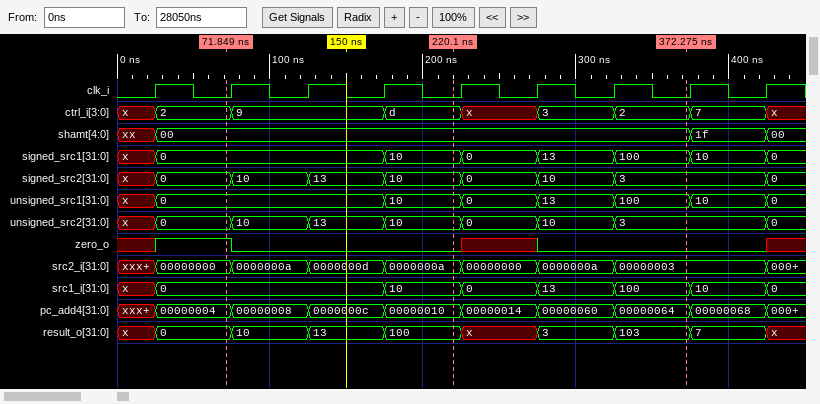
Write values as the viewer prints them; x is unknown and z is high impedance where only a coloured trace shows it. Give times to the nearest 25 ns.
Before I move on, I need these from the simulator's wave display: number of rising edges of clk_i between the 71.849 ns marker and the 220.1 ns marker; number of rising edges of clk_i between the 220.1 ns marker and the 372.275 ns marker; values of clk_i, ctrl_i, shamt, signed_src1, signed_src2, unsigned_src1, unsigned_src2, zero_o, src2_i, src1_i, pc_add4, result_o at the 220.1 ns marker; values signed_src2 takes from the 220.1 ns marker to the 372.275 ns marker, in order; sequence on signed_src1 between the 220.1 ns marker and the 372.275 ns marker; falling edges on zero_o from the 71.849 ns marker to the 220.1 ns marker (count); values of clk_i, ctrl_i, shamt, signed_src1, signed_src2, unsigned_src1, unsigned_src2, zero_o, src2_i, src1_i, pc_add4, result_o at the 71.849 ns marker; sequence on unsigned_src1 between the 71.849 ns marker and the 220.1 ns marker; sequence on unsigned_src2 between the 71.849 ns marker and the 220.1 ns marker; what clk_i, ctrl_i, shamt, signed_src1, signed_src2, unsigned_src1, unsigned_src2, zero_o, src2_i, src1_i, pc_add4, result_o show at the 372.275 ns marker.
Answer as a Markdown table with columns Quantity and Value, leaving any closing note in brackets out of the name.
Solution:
| Quantity | Value |
|---|---|
| number of rising edges of clk_i between the 71.849 ns marker and the 220.1 ns marker | 3 |
| number of rising edges of clk_i between the 220.1 ns marker and the 372.275 ns marker | 3 |
| values of clk_i, ctrl_i, shamt, signed_src1, signed_src2, unsigned_src1, unsigned_src2, zero_o, src2_i, src1_i, pc_add4, result_o at the 220.1 ns marker | clk_i=0, ctrl_i=d, shamt=00, signed_src1=10, signed_src2=10, unsigned_src1=10, unsigned_src2=10, zero_o=0, src2_i=0000000a, src1_i=10, pc_add4=00000010, result_o=100 |
| values signed_src2 takes from the 220.1 ns marker to the 372.275 ns marker, in order | 10, 0, 10, 3 |
| sequence on signed_src1 between the 220.1 ns marker and the 372.275 ns marker | 10, 0, 13, 100 |
| falling edges on zero_o from the 71.849 ns marker to the 220.1 ns marker | 1 |
| values of clk_i, ctrl_i, shamt, signed_src1, signed_src2, unsigned_src1, unsigned_src2, zero_o, src2_i, src1_i, pc_add4, result_o at the 71.849 ns marker | clk_i=0, ctrl_i=2, shamt=00, signed_src1=0, signed_src2=0, unsigned_src1=0, unsigned_src2=0, zero_o=1, src2_i=00000000, src1_i=0, pc_add4=00000004, result_o=0 |
| sequence on unsigned_src1 between the 71.849 ns marker and the 220.1 ns marker | 0, 10 |
| sequence on unsigned_src2 between the 71.849 ns marker and the 220.1 ns marker | 0, 10, 13, 10 |
| what clk_i, ctrl_i, shamt, signed_src1, signed_src2, unsigned_src1, unsigned_src2, zero_o, src2_i, src1_i, pc_add4, result_o show at the 372.275 ns marker | clk_i=0, ctrl_i=2, shamt=00, signed_src1=100, signed_src2=3, unsigned_src1=100, unsigned_src2=3, zero_o=0, src2_i=00000003, src1_i=100, pc_add4=00000064, result_o=103 |
